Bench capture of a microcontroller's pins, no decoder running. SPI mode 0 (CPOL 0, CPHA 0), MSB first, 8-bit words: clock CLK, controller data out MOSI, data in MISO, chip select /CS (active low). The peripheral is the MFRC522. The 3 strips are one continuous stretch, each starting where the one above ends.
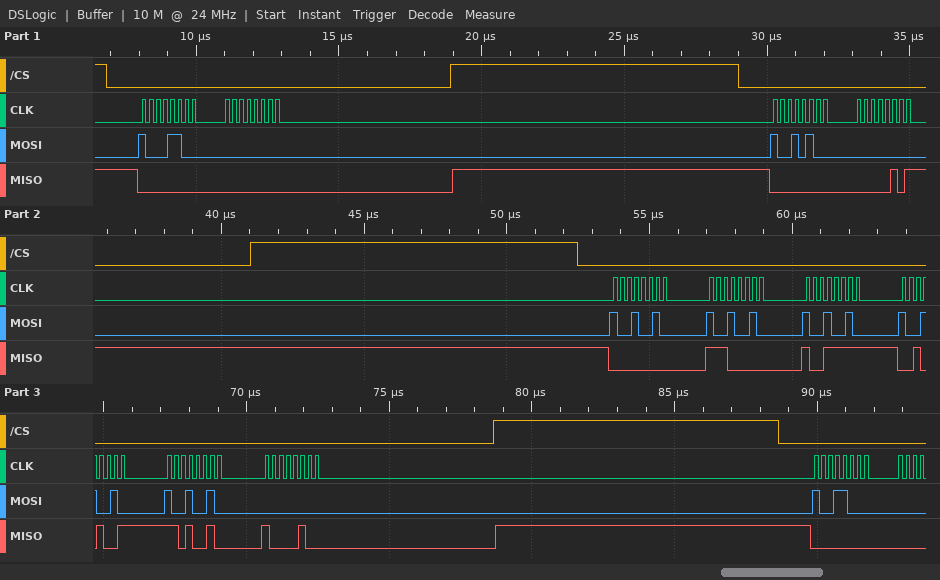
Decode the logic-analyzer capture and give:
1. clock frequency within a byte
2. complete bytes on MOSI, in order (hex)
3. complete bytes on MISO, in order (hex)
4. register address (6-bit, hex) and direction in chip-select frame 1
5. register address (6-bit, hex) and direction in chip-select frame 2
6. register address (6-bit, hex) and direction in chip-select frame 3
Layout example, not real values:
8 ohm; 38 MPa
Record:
4 MHz; 8C 00 94 00 92 92 92 92 92 00 98; 00 00 00 05 00 E0 9F 29 D2 84 00; 0x06 read; 0x0A read; 0x09 read
